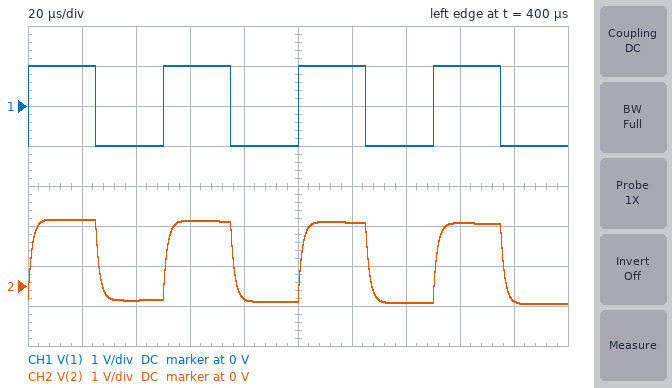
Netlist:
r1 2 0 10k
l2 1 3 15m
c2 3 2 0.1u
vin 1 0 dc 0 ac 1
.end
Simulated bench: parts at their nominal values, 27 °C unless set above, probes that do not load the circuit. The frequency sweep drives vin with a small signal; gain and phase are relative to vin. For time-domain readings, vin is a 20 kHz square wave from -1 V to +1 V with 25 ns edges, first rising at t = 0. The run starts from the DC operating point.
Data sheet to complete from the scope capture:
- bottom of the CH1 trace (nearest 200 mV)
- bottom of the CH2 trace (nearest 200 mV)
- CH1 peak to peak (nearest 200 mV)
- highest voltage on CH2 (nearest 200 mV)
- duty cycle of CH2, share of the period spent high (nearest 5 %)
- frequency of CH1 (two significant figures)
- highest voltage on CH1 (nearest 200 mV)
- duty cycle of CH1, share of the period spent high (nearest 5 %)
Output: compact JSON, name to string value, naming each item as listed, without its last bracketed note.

{"bottom of the CH1 trace": "-1.0 V", "bottom of the CH2 trace": "-400 mV", "CH1 peak to peak": "2.0 V", "highest voltage on CH2": "1.6 V", "duty cycle of CH2, share of the period spent high": "50 %", "frequency of CH1": "20 kHz", "highest voltage on CH1": "1.0 V", "duty cycle of CH1, share of the period spent high": "50 %"}
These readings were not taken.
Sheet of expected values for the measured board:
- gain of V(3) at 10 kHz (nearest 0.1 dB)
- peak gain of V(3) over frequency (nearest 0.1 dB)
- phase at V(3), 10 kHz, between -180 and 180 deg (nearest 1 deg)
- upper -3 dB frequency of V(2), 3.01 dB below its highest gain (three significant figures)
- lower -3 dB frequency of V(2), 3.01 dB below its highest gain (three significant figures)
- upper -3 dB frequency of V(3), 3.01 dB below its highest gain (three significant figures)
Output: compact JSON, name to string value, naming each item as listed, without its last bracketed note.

{"gain of V(3) at 10 kHz": "0 dB", "peak gain of V(3) over frequency": "0 dB", "phase at V(3), 10 kHz, between -180 and 180 deg": "-5 deg", "upper -3 dB frequency of V(2), 3.01 dB below its highest gain": "106 kHz", "lower -3 dB frequency of V(2), 3.01 dB below its highest gain": "159 Hz", "upper -3 dB frequency of V(3), 3.01 dB below its highest gain": "106 kHz"}
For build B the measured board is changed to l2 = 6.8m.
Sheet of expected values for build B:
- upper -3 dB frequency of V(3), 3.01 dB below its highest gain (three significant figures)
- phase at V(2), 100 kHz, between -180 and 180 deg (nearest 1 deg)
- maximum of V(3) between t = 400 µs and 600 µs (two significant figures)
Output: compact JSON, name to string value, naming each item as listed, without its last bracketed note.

{"upper -3 dB frequency of V(3), 3.01 dB below its highest gain": "234 kHz", "phase at V(2), 100 kHz, between -180 and 180 deg": "-23 deg", "maximum of V(3) between t = 400 µs and 600 µs": "1.0 V"}
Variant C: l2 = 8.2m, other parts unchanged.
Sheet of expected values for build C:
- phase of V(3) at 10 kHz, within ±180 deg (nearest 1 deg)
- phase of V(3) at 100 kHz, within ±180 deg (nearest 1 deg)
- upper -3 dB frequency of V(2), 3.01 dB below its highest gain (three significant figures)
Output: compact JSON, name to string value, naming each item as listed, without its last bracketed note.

{"phase of V(3) at 10 kHz, within ±180 deg": "-3 deg", "phase of V(3) at 100 kHz, within ±180 deg": "-27 deg", "upper -3 dB frequency of V(2), 3.01 dB below its highest gain": "194 kHz"}
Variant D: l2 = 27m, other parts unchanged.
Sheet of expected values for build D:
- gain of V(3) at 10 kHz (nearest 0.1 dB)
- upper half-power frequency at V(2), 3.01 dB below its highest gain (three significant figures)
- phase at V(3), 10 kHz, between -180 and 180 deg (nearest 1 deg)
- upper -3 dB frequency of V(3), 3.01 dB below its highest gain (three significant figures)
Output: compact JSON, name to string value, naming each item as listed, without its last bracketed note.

{"gain of V(3) at 10 kHz": "-0.1 dB", "upper half-power frequency at V(2), 3.01 dB below its highest gain": "59.1 kHz", "phase at V(3), 10 kHz, between -180 and 180 deg": "-10 deg", "upper -3 dB frequency of V(3), 3.01 dB below its highest gain": "58.8 kHz"}
